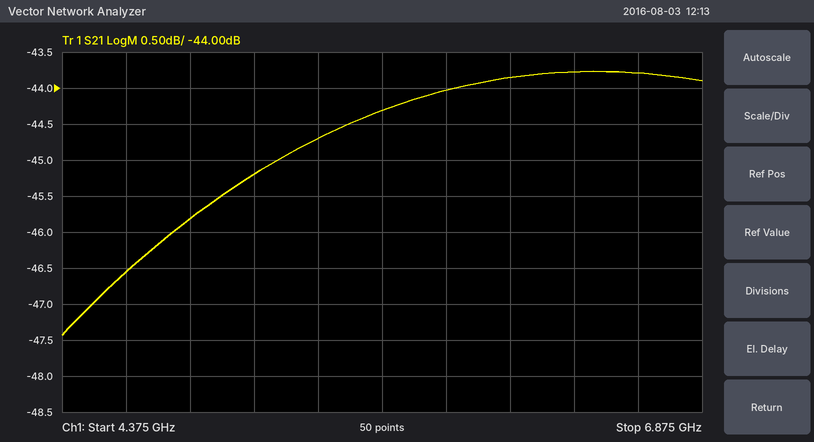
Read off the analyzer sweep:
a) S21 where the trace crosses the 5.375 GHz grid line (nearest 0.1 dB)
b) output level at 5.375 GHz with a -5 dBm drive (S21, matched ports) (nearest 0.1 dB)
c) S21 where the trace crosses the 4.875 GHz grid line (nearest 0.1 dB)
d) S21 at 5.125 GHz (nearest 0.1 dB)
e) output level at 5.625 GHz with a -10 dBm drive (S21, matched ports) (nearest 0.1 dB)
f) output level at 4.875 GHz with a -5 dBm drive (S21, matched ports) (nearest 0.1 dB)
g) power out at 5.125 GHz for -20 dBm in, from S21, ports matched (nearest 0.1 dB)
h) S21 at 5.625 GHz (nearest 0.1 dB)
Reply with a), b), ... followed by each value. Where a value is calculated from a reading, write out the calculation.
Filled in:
a) -44.7 dB
b) -5 dBm + (-44.7 dB) = -49.7 dBm
c) -45.8 dB
d) -45.2 dB
e) -10 dBm + (-44.3 dB) = -54.3 dBm
f) -5 dBm + (-45.8 dB) = -50.8 dBm
g) -20 dBm + (-45.2 dB) = -65.2 dBm
h) -44.3 dB
